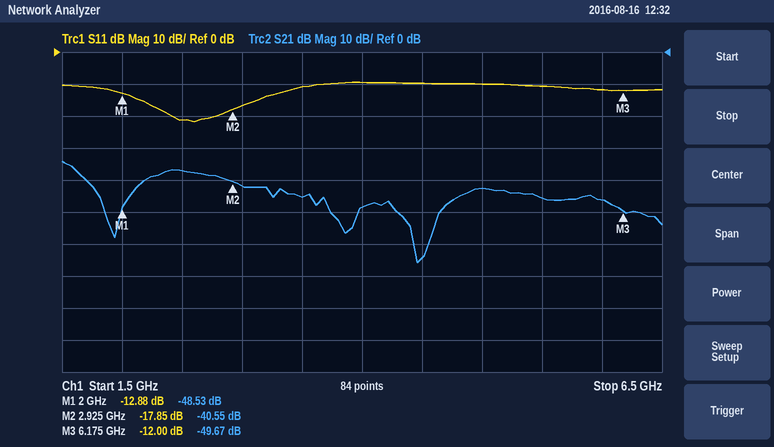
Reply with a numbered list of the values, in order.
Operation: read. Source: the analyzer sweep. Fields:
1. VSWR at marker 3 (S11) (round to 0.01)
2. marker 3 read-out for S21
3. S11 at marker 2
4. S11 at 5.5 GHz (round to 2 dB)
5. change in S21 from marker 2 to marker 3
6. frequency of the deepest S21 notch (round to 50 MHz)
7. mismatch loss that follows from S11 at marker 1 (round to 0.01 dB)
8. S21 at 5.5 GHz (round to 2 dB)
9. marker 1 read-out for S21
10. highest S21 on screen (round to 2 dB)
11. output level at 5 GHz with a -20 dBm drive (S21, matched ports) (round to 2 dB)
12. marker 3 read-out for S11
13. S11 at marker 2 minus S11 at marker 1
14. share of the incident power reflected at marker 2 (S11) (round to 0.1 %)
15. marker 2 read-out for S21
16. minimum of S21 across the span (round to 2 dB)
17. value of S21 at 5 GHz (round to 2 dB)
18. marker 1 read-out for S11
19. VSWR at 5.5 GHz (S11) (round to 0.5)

1. 1.67
2. -49.67 dB
3. -17.85 dB
4. -10 dB
5. -9.12 dB
6. 4.45 GHz
7. 0.23 dB
8. -46 dB
9. -48.53 dB
10. -34 dB
11. -62 dBm
12. -12.00 dB
13. -4.97 dB
14. 1.6 %
15. -40.55 dB
16. -66 dB
17. -42 dB
18. -12.88 dB
19. 2.0
